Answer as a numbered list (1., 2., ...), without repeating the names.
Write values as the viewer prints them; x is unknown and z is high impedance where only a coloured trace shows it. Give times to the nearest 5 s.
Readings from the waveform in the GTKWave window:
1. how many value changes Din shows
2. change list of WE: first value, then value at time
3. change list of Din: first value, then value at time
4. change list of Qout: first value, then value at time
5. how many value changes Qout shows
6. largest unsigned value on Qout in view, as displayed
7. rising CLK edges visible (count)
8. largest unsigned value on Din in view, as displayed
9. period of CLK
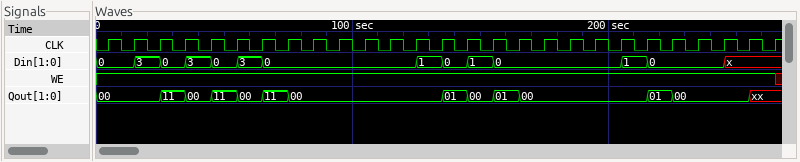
1. 13
2. 1, x at 265 s
3. 0, 3 at 15 s, 0 at 25 s, 3 at 35 s, 0 at 45 s, 3 at 55 s, 0 at 65 s, 1 at 125 s, 0 at 135 s, 1 at 145 s, 0 at 155 s, 1 at 205 s, 0 at 215 s, x at 245 s
4. 00, 11 at 25 s, 00 at 35 s, 11 at 45 s, 00 at 55 s, 11 at 65 s, 00 at 75 s, 01 at 135 s, 00 at 145 s, 01 at 155 s, 00 at 165 s, 01 at 215 s, 00 at 225 s, xx at 255 s
5. 13
6. 11
7. 27
8. 3
9. 10 s
